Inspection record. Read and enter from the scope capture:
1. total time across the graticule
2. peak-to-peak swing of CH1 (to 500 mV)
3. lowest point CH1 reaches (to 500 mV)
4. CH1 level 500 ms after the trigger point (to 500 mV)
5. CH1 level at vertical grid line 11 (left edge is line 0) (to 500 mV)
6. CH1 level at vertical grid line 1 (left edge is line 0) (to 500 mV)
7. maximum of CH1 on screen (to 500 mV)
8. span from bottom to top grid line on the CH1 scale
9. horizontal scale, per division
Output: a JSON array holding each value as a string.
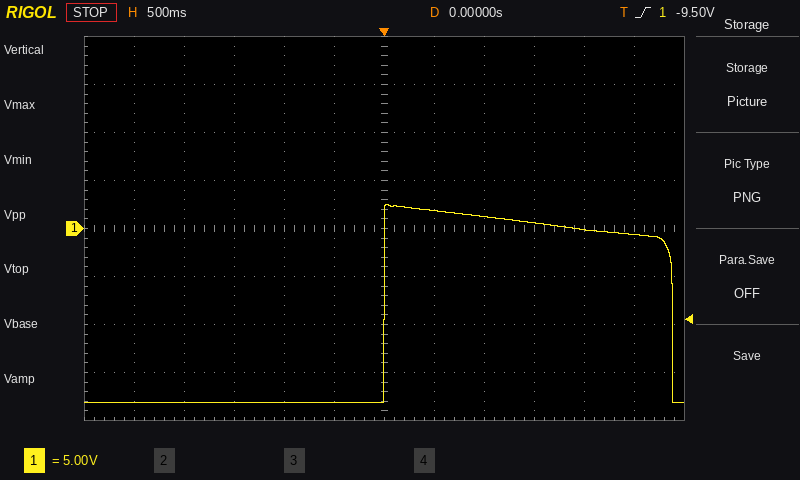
["6 s", "20.5 V", "-18.0 V", "2.0 V", "-500 mV", "-18.0 V", "2.5 V", "40 V", "500 ms"]
